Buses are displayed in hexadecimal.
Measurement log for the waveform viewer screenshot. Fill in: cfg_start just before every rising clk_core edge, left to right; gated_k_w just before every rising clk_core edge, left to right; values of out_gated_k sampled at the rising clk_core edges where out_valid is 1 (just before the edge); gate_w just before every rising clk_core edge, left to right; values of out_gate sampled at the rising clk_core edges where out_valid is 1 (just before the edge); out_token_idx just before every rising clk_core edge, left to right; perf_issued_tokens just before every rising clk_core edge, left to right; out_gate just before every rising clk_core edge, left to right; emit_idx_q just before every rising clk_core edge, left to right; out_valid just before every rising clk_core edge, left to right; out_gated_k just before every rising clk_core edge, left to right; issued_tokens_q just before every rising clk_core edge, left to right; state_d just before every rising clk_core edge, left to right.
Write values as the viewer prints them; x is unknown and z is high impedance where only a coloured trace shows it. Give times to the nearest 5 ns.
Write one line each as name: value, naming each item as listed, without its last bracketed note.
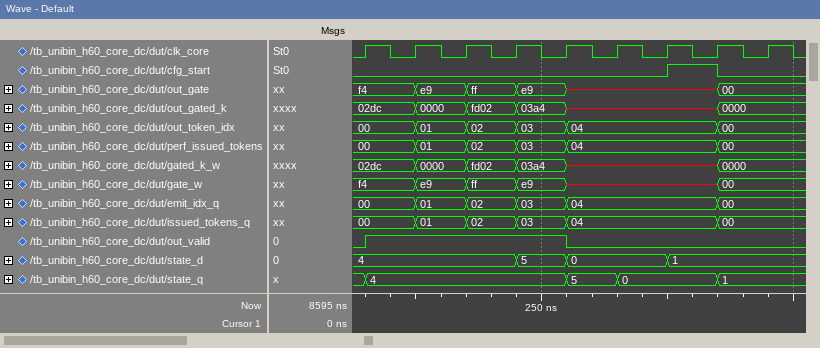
cfg_start just before every rising clk_core edge, left to right: 0 0 0 0 0 0 0 1 0
gated_k_w just before every rising clk_core edge, left to right: 02dc, 02dc, 0000, fd02, 03a4, x, x, x, 0000
values of out_gated_k sampled at the rising clk_core edges where out_valid is 1: 02dc, 0000, fd02, 03a4
gate_w just before every rising clk_core edge, left to right: f4, f4, e9, ff, e9, x, x, x, 00
values of out_gate sampled at the rising clk_core edges where out_valid is 1: f4, e9, ff, e9
out_token_idx just before every rising clk_core edge, left to right: 00, 00, 01, 02, 03, 04, 04, 04, 00
perf_issued_tokens just before every rising clk_core edge, left to right: 00, 00, 01, 02, 03, 04, 04, 04, 00
out_gate just before every rising clk_core edge, left to right: f4, f4, e9, ff, e9, x, x, x, 00
emit_idx_q just before every rising clk_core edge, left to right: 00, 00, 01, 02, 03, 04, 04, 04, 00
out_valid just before every rising clk_core edge, left to right: 0 1 1 1 1 0 0 0 0
out_gated_k just before every rising clk_core edge, left to right: 02dc, 02dc, 0000, fd02, 03a4, x, x, x, 0000
issued_tokens_q just before every rising clk_core edge, left to right: 00, 00, 01, 02, 03, 04, 04, 04, 00
state_d just before every rising clk_core edge, left to right: 4, 4, 4, 4, 5, 0, 0, 1, 1
